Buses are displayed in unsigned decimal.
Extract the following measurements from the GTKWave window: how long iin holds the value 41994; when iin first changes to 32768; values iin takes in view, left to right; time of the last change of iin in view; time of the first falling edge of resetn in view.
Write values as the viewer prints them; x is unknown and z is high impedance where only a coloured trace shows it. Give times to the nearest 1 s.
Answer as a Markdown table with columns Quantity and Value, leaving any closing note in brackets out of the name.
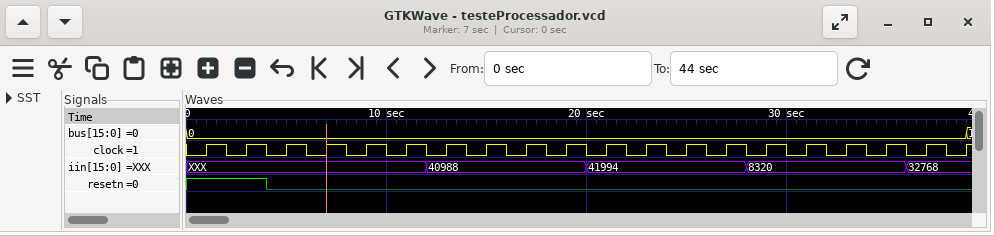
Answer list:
| Quantity | Value |
|---|---|
| how long iin holds the value 41994 | 8 s |
| when iin first changes to 32768 | 36 s |
| values iin takes in view, left to right | XXX, 40988, 41994, 8320, 32768 |
| time of the last change of iin in view | 36 s |
| time of the first falling edge of resetn in view | 4 s |
